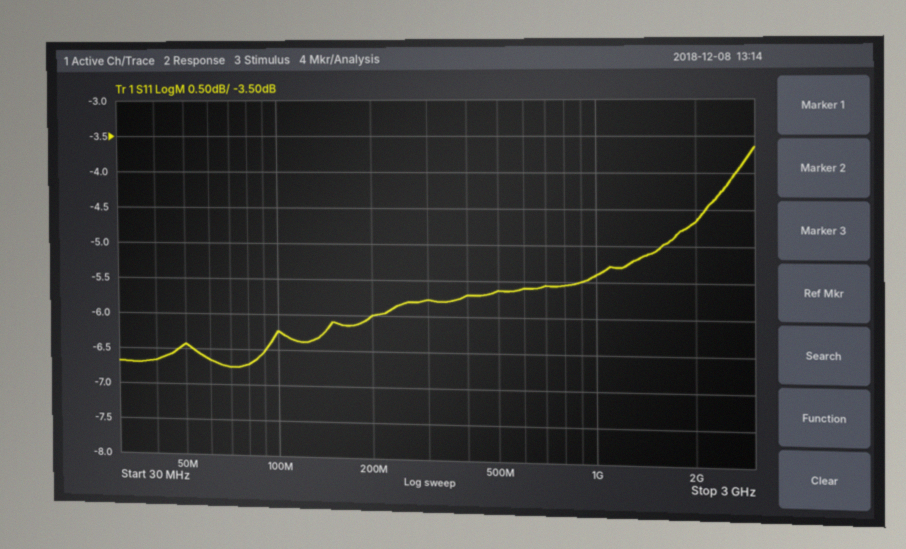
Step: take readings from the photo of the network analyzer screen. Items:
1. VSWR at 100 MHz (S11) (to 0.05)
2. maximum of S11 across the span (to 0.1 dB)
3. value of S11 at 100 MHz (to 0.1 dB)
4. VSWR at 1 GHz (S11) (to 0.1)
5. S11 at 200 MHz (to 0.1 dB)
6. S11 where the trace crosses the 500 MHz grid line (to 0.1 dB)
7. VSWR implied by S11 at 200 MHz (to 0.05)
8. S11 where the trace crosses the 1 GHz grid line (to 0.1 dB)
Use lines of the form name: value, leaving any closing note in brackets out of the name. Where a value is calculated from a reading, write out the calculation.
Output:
VSWR at 100 MHz (S11): |Γ| = 10^(-6.2/20) = 0.4898; VSWR = (1 + 0.4898)/(1 − 0.4898) ≈ 2.92, so 2.90 to the nearest 0.05
maximum of S11 across the span: -3.6 dB
value of S11 at 100 MHz: -6.2 dB
VSWR at 1 GHz (S11): |Γ| = 10^(-5.4/20) = 0.5370; VSWR = (1 + 0.5370)/(1 − 0.5370) ≈ 3.3
S11 at 200 MHz: -6.0 dB
S11 where the trace crosses the 500 MHz grid line: -5.6 dB
VSWR implied by S11 at 200 MHz: |Γ| = 10^(-6/20) = 0.5012; VSWR = (1 + 0.5012)/(1 − 0.5012) ≈ 3.01, so 3.00 to the nearest 0.05
S11 where the trace crosses the 1 GHz grid line: -5.4 dB
